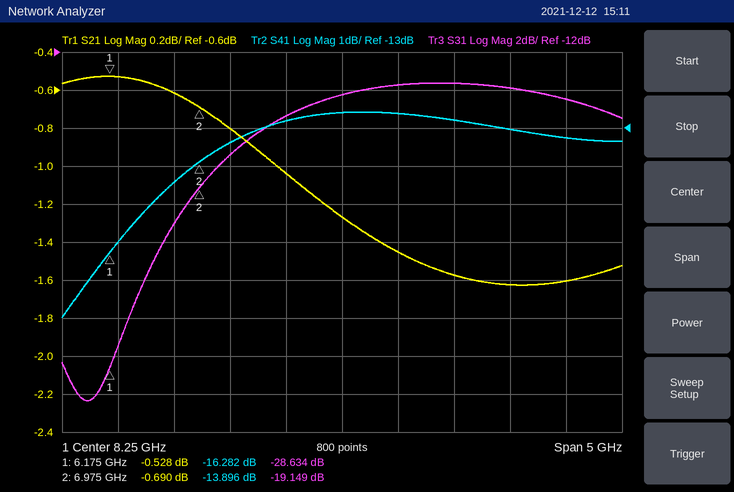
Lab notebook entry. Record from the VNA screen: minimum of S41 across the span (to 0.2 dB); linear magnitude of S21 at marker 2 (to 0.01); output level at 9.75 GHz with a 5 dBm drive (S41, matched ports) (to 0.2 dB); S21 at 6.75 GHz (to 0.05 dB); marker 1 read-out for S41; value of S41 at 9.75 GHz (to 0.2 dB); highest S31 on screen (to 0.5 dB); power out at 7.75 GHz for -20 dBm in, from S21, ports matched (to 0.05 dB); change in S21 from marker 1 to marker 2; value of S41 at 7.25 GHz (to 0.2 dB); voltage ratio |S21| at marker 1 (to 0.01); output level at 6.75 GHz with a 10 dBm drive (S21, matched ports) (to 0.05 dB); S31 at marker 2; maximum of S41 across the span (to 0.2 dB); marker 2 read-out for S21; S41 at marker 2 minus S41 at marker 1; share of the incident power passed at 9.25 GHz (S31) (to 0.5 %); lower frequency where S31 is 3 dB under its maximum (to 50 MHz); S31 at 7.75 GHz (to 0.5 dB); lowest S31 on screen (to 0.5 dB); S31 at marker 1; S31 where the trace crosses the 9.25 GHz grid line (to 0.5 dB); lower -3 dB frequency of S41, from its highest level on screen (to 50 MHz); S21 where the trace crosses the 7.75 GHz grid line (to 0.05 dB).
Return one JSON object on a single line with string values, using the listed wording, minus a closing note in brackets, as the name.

{"minimum of S41 across the span": "-18.0 dB", "linear magnitude of S21 at marker 2": "0.92", "output level at 9.75 GHz with a 5 dBm drive (S41, matched ports)": "-8.0 dBm", "S21 at 6.75 GHz": "-0.60 dB", "marker 1 read-out for S41": "-16.282 dB", "value of S41 at 9.75 GHz": "-13.0 dB", "highest S31 on screen": "-13.5 dB", "power out at 7.75 GHz for -20 dBm in, from S21, ports matched": "-21.05 dBm", "change in S21 from marker 1 to marker 2": "-0.162 dB", "value of S41 at 7.25 GHz": "-13.4 dB", "voltage ratio |S21| at marker 1": "0.94", "output level at 6.75 GHz with a 10 dBm drive (S21, matched ports)": "9.40 dBm", "S31 at marker 2": "-19.149 dB", "maximum of S41 across the span": "-12.6 dB", "marker 2 read-out for S21": "-0.690 dB", "S41 at marker 2 minus S41 at marker 1": "2.386 dB", "share of the incident power passed at 9.25 GHz (S31)": "4.5 %", "lower frequency where S31 is 3 dB under its maximum": "7.40 GHz", "S31 at 7.75 GHz": "-15.5 dB", "lowest S31 on screen": "-30.5 dB", "S31 at marker 1": "-28.634 dB", "S31 where the trace crosses the 9.25 GHz grid line": "-13.5 dB", "lower -3 dB frequency of S41, from its highest level on screen": "6.35 GHz", "S21 where the trace crosses the 7.75 GHz grid line": "-1.05 dB"}
